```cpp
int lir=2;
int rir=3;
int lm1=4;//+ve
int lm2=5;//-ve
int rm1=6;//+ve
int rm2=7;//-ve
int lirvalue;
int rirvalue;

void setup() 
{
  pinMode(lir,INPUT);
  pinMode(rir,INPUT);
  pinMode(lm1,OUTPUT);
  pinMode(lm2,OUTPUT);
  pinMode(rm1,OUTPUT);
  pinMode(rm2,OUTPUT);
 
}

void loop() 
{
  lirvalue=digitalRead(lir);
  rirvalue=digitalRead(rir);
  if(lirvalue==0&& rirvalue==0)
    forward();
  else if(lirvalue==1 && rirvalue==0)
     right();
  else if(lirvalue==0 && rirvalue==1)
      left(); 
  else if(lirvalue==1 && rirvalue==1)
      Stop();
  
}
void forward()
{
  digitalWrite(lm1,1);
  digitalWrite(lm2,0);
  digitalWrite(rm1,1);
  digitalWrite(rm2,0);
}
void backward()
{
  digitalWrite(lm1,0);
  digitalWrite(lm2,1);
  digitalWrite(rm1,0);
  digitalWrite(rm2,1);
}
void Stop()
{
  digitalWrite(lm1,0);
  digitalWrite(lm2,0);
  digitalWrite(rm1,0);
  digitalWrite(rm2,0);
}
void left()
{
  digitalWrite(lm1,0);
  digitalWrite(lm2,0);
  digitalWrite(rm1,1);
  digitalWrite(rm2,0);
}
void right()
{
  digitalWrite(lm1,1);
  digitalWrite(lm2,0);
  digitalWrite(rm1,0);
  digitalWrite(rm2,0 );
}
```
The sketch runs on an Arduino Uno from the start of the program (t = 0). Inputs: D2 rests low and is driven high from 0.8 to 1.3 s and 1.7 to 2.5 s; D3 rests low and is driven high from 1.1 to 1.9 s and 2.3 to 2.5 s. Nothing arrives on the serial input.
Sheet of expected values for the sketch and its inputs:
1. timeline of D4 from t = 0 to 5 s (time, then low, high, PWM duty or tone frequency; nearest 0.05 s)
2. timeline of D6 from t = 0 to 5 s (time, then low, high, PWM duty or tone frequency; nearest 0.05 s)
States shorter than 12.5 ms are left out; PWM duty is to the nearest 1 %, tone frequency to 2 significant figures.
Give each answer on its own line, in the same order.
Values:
0 s high; 1.1 s low; 1.9 s high; 2.3 s low; 2.5 s high
0 s high; 0.8 s low; 1.3 s high; 1.7 s low; 2.5 s high
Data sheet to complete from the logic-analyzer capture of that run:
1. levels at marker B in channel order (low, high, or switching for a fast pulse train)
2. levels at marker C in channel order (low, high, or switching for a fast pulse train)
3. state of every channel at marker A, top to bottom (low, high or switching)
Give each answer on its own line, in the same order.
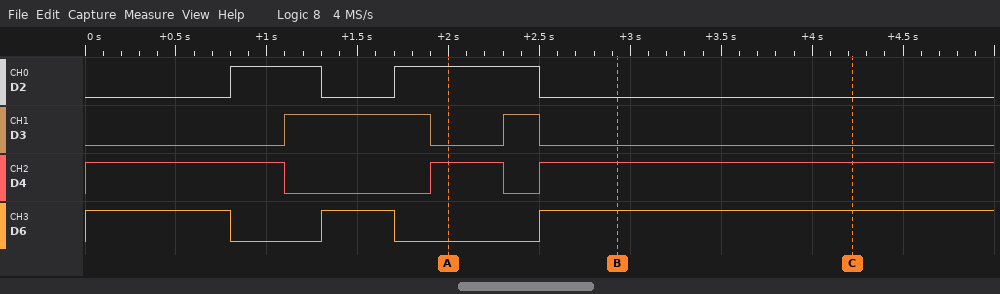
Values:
D2 low, D3 low, D4 high, D6 high
D2 low, D3 low, D4 high, D6 high
D2 high, D3 low, D4 high, D6 low
